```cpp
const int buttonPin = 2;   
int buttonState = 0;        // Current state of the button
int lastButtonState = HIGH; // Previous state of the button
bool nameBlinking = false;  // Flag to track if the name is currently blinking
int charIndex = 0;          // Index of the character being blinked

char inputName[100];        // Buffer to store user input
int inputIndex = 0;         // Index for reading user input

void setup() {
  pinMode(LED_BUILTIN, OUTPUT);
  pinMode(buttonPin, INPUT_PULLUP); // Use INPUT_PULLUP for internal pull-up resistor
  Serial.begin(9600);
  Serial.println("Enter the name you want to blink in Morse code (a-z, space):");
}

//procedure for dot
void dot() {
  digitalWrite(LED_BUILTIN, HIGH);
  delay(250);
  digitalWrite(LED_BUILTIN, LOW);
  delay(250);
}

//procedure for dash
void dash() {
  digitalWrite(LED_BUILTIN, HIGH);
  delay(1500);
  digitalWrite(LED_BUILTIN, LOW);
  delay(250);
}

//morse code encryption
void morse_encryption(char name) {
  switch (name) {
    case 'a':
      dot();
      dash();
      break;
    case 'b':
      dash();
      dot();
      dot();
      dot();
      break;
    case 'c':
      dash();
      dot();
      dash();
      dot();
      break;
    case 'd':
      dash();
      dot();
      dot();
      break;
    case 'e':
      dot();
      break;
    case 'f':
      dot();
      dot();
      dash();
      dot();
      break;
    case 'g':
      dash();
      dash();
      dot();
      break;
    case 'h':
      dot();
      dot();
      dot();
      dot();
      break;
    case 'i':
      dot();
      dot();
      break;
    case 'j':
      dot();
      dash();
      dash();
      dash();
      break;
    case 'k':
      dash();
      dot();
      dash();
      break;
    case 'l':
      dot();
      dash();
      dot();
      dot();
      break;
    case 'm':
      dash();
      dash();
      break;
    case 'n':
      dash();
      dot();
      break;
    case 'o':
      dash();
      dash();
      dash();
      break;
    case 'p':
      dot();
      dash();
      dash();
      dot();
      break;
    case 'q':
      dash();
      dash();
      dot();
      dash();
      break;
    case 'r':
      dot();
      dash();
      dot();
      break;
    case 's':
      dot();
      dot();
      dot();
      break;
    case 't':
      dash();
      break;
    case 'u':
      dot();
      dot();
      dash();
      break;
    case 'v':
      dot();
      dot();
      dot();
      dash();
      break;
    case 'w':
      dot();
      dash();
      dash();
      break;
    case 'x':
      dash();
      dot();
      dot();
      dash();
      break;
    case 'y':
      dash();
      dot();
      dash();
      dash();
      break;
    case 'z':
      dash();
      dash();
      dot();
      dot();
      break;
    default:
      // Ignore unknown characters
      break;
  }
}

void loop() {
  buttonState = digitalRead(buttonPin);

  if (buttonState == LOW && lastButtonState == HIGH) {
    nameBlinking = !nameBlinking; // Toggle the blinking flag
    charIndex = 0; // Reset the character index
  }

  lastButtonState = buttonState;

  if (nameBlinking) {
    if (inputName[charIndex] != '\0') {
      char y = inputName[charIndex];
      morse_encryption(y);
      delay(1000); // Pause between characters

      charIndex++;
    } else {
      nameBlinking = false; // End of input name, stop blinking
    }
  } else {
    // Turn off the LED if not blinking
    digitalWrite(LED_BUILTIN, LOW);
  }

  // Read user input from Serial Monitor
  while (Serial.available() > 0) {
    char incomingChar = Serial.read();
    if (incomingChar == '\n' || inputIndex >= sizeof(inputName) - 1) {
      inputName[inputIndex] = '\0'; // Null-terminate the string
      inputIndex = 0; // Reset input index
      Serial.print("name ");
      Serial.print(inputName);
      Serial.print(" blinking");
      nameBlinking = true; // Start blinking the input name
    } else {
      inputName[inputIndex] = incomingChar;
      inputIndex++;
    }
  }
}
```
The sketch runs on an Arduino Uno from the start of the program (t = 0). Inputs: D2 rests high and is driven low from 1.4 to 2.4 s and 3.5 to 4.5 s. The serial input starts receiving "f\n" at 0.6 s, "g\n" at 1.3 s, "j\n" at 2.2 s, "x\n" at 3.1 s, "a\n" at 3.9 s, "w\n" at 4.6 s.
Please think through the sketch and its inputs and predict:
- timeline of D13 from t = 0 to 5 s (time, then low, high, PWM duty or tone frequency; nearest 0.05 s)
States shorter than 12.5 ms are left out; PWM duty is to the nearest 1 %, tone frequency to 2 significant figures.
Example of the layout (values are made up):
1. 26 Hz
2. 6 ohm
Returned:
1. 0 s low; 0.6 s high; 0.85 s low; 1.1 s high; 1.35 s low; 1.6 s high; 3.1 s low; 3.35 s high; 3.6 s low
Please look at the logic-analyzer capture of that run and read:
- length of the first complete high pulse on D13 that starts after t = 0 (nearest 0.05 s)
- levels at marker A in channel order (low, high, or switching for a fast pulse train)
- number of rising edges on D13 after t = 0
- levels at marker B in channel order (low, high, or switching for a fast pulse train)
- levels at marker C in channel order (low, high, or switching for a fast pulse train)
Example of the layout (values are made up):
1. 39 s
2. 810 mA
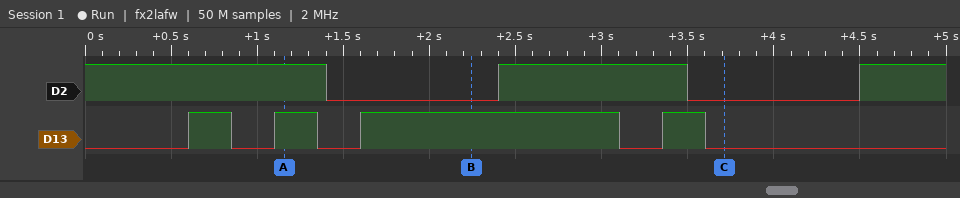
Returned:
1. 0.25 s
2. D2 high, D13 high
3. 4
4. D2 low, D13 high
5. D2 low, D13 low
